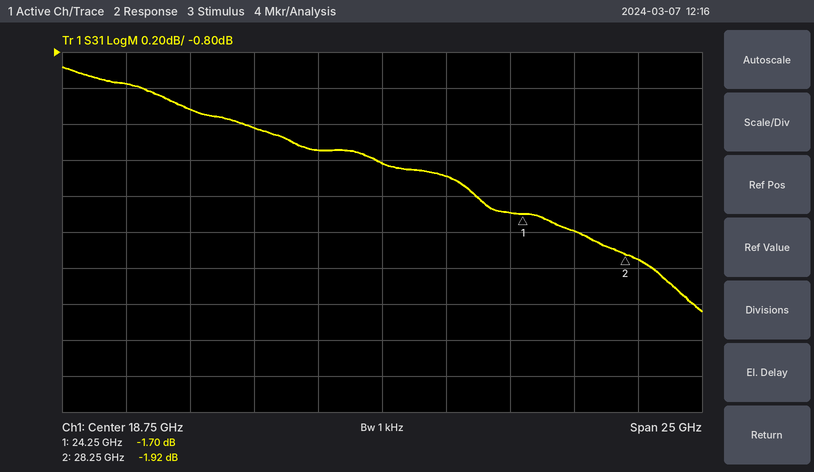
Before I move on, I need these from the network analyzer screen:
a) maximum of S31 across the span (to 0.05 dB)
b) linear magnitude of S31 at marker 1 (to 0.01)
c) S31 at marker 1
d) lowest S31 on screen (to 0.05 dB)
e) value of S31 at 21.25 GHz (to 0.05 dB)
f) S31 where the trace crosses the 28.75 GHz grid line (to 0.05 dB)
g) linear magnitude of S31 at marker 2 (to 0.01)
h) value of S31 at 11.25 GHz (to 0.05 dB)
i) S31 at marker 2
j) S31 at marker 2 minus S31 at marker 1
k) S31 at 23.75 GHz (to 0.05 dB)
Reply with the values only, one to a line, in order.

-0.90 dB
0.82
-1.70 dB
-2.25 dB
-1.50 dB
-1.95 dB
0.80
-1.10 dB
-1.92 dB
-0.22 dB
-1.70 dB
